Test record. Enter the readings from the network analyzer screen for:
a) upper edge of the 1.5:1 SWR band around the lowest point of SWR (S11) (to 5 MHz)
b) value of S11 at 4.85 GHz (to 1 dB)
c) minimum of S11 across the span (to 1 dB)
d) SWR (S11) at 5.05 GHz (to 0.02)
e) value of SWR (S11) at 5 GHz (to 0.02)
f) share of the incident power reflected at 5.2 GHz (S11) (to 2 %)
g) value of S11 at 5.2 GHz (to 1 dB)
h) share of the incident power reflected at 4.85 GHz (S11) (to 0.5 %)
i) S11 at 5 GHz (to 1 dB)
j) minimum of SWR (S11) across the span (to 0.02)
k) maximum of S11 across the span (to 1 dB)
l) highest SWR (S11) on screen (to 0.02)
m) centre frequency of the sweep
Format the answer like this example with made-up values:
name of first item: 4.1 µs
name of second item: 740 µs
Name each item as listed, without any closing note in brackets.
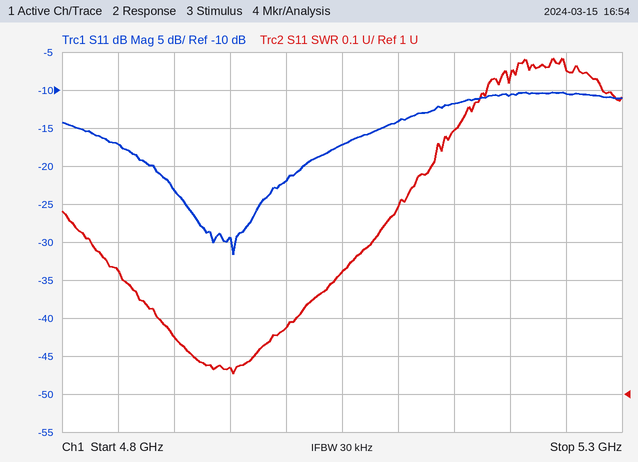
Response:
upper edge of the 1.5:1 SWR band around the lowest point of SWR (S11): 5.100 GHz
value of S11 at 4.85 GHz: -17 dB
minimum of S11 across the span: -32 dB
SWR (S11) at 5.05 GHz: 1.32
value of SWR (S11) at 5 GHz: 1.18
share of the incident power reflected at 5.2 GHz (S11): 8 %
value of S11 at 5.2 GHz: -11 dB
share of the incident power reflected at 4.85 GHz (S11): 2.0 %
S11 at 5 GHz: -22 dB
minimum of SWR (S11) across the span: 1.06
maximum of S11 across the span: -10 dB
highest SWR (S11) on screen: 1.88
centre frequency of the sweep: 5.05 GHz
